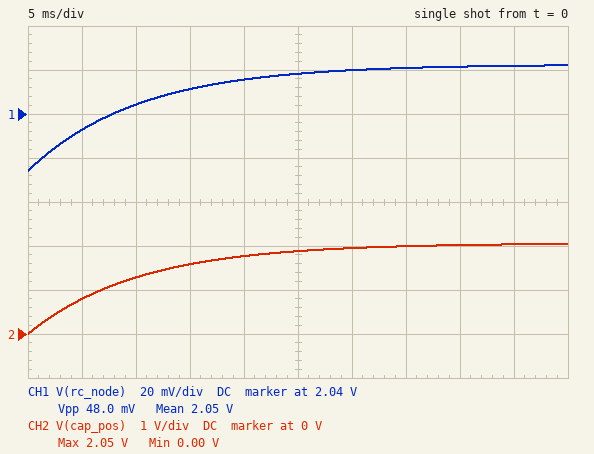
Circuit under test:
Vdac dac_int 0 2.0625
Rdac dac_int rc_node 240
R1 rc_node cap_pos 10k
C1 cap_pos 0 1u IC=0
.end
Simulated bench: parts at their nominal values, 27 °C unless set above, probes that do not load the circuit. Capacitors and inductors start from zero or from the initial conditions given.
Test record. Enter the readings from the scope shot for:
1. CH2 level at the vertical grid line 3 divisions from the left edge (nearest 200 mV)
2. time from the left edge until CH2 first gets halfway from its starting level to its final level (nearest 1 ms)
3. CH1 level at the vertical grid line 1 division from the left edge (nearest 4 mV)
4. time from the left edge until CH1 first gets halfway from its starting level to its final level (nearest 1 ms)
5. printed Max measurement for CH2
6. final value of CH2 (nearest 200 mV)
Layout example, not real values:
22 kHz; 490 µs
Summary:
1.6 V; 7 ms; 2.032 V; 7 ms; 2.05 V; 2.0 V
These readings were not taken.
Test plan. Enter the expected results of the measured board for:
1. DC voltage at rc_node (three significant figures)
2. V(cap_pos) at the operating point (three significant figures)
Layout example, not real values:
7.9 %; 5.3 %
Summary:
2.06 V; 2.06 V
